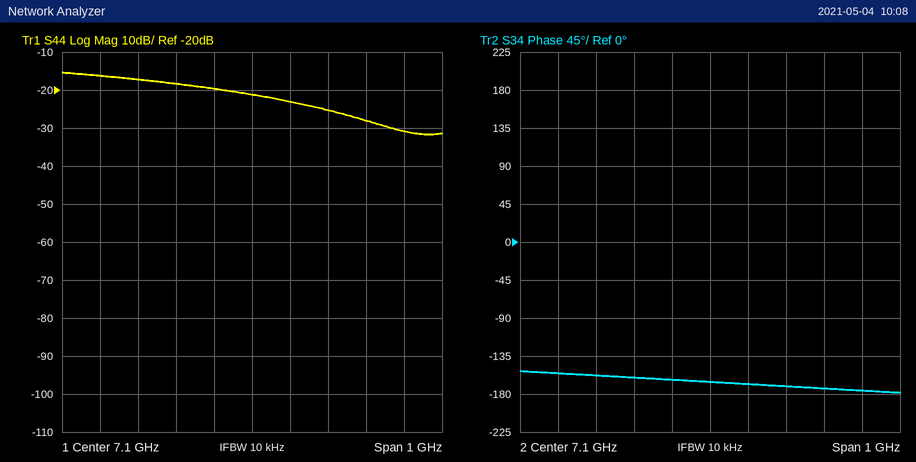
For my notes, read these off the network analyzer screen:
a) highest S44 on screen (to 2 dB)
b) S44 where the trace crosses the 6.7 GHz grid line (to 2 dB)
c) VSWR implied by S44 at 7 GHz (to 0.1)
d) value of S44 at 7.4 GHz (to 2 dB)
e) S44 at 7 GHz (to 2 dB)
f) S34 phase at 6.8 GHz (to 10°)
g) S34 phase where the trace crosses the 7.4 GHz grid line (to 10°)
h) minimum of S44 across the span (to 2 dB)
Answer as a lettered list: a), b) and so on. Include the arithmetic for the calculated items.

a) -16 dB
b) -16 dB
c) |Γ| = 10^(-20/20) = 0.1000; VSWR = (1 + 0.1000)/(1 − 0.1000) ≈ 1.2
d) -28 dB
e) -20 dB
f) -160°
g) -170°
h) -32 dB
